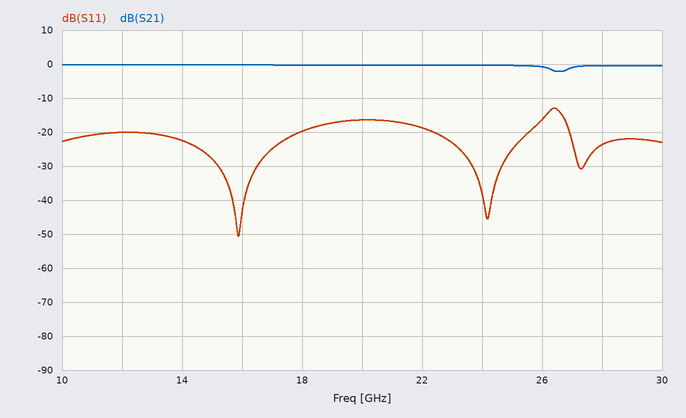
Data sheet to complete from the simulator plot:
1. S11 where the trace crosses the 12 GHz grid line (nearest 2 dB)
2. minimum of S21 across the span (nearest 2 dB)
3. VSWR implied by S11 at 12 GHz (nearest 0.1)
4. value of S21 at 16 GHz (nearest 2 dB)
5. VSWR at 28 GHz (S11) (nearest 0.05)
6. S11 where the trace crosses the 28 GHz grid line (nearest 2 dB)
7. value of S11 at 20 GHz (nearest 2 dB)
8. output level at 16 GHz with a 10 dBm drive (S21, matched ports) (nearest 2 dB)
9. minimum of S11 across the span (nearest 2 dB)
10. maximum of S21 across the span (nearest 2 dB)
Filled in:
-20 dB
-2 dB
1.2
0 dB
1.15
-24 dB
-16 dB
10 dBm
-50 dB
0 dB
